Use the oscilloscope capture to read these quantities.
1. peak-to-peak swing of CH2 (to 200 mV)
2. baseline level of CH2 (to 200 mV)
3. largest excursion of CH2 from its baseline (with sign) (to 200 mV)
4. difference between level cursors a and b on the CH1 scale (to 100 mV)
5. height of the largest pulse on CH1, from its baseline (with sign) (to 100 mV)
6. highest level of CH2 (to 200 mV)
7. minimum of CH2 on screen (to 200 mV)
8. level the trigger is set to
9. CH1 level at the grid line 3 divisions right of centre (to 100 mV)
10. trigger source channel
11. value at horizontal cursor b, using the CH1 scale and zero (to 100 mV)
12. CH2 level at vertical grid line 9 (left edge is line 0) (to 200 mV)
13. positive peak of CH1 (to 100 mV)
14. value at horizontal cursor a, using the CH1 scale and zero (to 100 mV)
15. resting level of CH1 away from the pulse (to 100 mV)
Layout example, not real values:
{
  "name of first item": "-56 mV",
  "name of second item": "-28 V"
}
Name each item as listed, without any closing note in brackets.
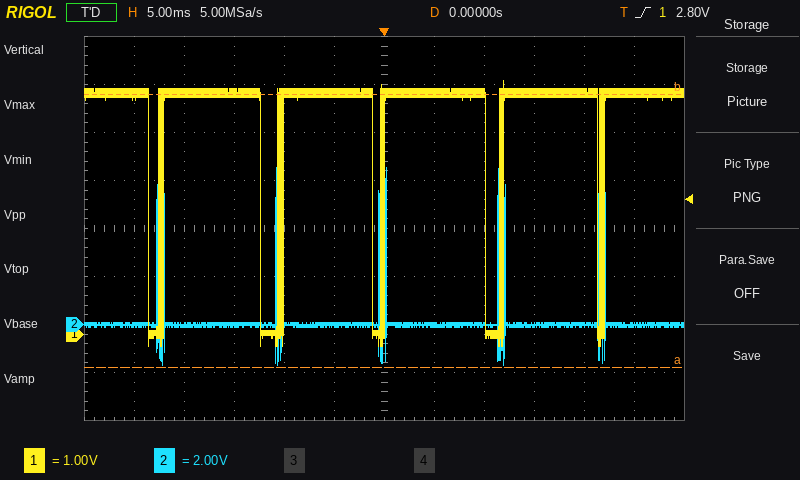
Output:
{
  "peak-to-peak swing of CH2": "8.2 V",
  "baseline level of CH2": "0.0 V",
  "largest excursion of CH2 from its baseline (with sign)": "+6.6 V",
  "difference between level cursors a and b on the CH1 scale": "5.7 V",
  "height of the largest pulse on CH1, from its baseline (with sign)": "-5.3 V",
  "highest level of CH2": "6.6 V",
  "minimum of CH2 on screen": "-1.6 V",
  "level the trigger is set to": "2.80 V",
  "CH1 level at the grid line 3 divisions right of centre": "5.0 V",
  "trigger source channel": "CH1",
  "value at horizontal cursor b, using the CH1 scale and zero": "5.0 V",
  "CH2 level at vertical grid line 9 (left edge is line 0)": "0.0 V",
  "positive peak of CH1": "5.3 V",
  "value at horizontal cursor a, using the CH1 scale and zero": "-700 mV",
  "resting level of CH1 away from the pulse": "5.0 V"
}
